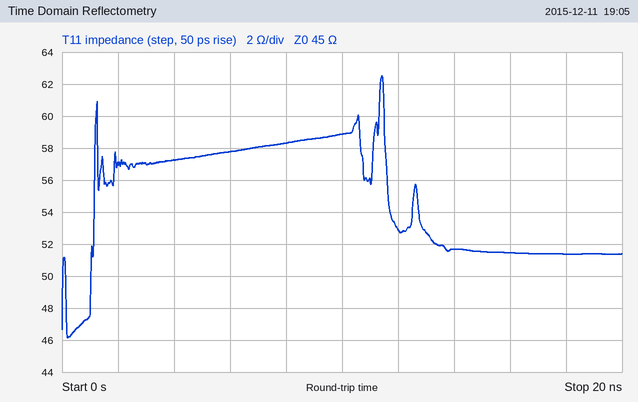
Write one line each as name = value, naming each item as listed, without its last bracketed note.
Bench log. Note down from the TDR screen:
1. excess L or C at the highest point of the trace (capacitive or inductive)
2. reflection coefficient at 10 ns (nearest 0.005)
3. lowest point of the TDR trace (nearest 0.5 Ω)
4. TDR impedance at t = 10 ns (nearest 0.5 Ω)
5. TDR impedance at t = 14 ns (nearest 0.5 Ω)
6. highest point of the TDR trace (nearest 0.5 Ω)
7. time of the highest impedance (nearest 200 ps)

excess L or C at the highest point of the trace = inductive
reflection coefficient at 10 ns = +0.135
lowest point of the TDR trace = 46.0 Ω
TDR impedance at t = 10 ns = 59.0 Ω
TDR impedance at t = 14 ns = 51.5 Ω
highest point of the TDR trace = 62.5 Ω
time of the highest impedance = 11.4 ns
